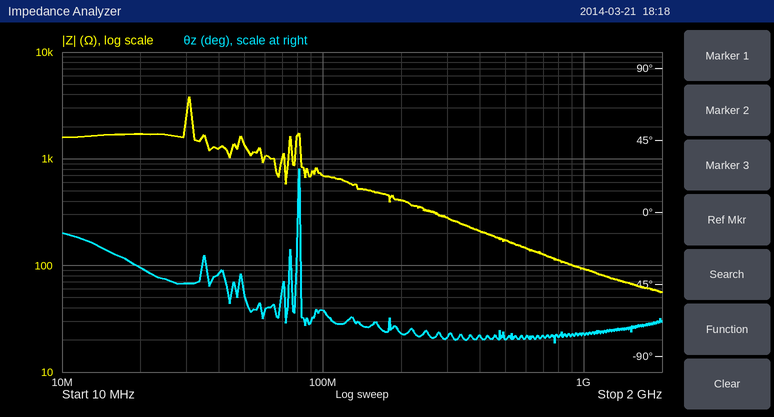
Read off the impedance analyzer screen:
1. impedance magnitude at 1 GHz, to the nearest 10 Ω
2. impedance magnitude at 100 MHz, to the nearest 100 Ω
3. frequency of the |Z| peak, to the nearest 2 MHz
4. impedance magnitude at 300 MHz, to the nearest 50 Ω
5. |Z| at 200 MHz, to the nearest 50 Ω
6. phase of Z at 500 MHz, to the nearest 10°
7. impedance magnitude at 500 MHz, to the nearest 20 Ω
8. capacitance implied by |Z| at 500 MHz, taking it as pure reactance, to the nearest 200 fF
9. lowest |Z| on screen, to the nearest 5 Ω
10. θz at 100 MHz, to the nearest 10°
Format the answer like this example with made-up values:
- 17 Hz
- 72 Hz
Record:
- 90 Ω
- 700 Ω
- 30 MHz
- 300 Ω
- 400 Ω
- -80°
- 180 Ω
- 1.8 pF
- 55 Ω
- -60°
